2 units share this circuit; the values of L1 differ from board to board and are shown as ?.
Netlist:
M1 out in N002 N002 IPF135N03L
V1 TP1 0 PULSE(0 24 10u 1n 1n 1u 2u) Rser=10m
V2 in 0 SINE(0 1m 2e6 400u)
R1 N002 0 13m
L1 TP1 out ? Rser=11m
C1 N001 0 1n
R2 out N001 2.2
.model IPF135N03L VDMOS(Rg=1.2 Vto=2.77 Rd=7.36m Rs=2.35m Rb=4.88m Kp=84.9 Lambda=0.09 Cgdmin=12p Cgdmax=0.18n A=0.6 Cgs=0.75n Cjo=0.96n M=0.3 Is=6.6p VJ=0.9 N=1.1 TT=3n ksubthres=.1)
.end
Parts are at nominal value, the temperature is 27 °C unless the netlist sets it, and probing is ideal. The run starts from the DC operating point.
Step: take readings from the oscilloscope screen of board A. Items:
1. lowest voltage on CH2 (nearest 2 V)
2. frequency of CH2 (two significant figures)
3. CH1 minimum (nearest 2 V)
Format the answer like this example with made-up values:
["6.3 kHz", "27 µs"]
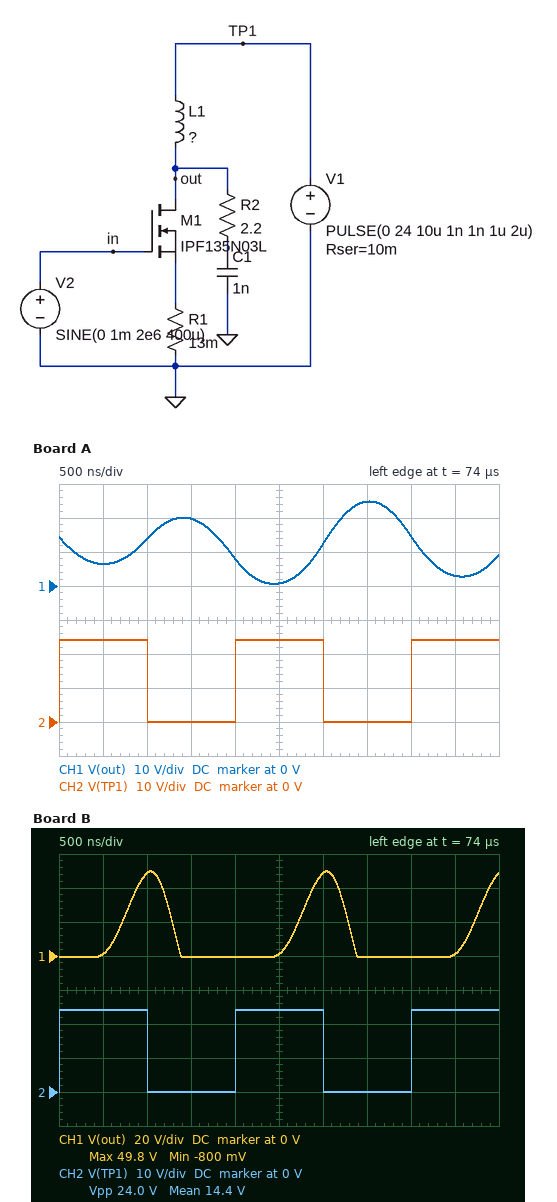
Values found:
["0 V", "500 kHz", "0 V"]
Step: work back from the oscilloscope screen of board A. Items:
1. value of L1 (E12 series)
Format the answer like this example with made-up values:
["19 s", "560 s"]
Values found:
["180 µH"]
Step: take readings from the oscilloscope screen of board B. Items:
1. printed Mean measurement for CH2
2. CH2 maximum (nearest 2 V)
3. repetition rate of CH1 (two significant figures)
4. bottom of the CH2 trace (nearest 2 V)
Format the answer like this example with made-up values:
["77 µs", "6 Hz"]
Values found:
["14.4 V", "24 V", "500 kHz", "0 V"]
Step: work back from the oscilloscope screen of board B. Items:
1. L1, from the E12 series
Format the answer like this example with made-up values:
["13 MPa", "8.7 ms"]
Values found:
["33 µH"]
